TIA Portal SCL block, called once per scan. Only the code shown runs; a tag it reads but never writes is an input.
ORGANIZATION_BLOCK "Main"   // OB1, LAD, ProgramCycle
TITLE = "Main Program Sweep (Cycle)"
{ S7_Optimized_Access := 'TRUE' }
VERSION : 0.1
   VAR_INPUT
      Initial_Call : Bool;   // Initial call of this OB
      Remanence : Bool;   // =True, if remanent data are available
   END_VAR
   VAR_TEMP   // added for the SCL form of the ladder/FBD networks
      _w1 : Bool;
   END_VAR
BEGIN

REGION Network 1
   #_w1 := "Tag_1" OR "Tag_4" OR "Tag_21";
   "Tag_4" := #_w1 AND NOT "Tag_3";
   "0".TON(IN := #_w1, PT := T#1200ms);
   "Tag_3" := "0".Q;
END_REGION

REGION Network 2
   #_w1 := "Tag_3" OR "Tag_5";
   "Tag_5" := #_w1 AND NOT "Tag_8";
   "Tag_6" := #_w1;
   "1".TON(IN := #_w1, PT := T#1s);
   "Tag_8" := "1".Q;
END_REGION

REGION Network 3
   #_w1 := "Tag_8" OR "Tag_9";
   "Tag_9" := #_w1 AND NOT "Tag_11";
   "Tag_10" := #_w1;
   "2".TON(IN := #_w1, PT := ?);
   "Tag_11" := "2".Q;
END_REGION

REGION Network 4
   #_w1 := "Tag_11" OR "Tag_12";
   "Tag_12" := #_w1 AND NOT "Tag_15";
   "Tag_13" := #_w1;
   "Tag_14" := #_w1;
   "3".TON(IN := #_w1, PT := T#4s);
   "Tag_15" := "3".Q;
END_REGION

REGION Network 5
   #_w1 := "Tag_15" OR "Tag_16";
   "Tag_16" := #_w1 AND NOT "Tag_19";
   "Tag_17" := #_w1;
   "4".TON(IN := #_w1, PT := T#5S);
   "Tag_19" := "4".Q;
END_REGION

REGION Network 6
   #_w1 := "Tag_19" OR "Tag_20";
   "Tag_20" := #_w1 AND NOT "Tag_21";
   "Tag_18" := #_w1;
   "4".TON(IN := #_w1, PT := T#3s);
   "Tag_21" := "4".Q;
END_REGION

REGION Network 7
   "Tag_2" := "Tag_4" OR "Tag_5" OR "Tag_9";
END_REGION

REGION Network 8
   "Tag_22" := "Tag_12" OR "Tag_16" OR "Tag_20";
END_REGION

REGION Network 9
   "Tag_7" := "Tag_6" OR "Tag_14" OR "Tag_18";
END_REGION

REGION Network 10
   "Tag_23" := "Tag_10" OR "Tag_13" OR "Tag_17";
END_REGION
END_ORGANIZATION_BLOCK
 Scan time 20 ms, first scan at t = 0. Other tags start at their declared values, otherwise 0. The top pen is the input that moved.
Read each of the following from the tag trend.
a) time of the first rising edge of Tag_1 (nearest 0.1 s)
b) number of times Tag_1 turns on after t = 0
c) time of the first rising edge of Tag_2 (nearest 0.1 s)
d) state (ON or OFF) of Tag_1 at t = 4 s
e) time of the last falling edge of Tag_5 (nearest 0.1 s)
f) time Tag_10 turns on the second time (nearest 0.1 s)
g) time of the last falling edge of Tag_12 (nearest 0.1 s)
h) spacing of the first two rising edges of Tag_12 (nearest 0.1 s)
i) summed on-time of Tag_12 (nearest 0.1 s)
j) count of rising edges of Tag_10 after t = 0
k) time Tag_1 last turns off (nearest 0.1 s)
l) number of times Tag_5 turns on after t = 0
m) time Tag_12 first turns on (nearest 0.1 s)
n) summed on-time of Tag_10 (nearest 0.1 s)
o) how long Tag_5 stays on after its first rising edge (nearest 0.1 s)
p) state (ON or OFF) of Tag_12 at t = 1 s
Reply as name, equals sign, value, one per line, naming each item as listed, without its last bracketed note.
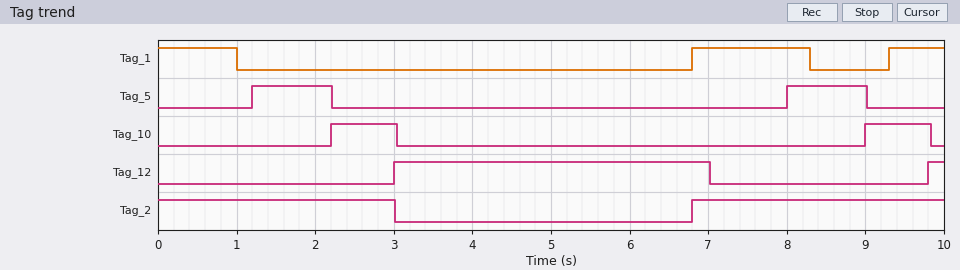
time of the first rising edge of Tag_1 = 6.8 s
number of times Tag_1 turns on after t = 0 = 2
time of the first rising edge of Tag_2 = 6.8 s
state (ON or OFF) of Tag_1 at t = 4 s = OFF
time of the last falling edge of Tag_5 = 9.0 s
time Tag_10 turns on the second time = 9.0 s
time of the last falling edge of Tag_12 = 7.0 s
spacing of the first two rising edges of Tag_12 = 6.8 s
summed on-time of Tag_12 = 4.2 s
count of rising edges of Tag_10 after t = 0 = 2
time Tag_1 last turns off = 8.3 s
number of times Tag_5 turns on after t = 0 = 2
time Tag_12 first turns on = 3.0 s
summed on-time of Tag_10 = 1.7 s
how long Tag_5 stays on after its first rising edge = 1.0 s
state (ON or OFF) of Tag_12 at t = 1 s = OFF
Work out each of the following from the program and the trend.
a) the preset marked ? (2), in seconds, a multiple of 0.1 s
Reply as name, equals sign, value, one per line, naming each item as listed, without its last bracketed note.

the preset marked ? (2), in seconds, a multiple of 0.1 s = 0.8 s
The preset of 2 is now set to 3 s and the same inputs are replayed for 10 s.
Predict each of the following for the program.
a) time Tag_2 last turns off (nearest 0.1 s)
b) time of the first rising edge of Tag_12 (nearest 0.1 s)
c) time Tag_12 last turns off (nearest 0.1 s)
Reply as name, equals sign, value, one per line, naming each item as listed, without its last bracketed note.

time Tag_2 last turns off = 5.2 s
time of the first rising edge of Tag_12 = 5.2 s
time Tag_12 last turns off = 9.2 s
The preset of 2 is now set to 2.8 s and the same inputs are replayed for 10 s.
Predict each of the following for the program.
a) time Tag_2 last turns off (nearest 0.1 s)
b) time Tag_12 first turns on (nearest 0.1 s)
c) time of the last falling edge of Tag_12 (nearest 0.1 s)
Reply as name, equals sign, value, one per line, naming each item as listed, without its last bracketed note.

time Tag_2 last turns off = 5.0 s
time Tag_12 first turns on = 5.0 s
time of the last falling edge of Tag_12 = 9.0 s
